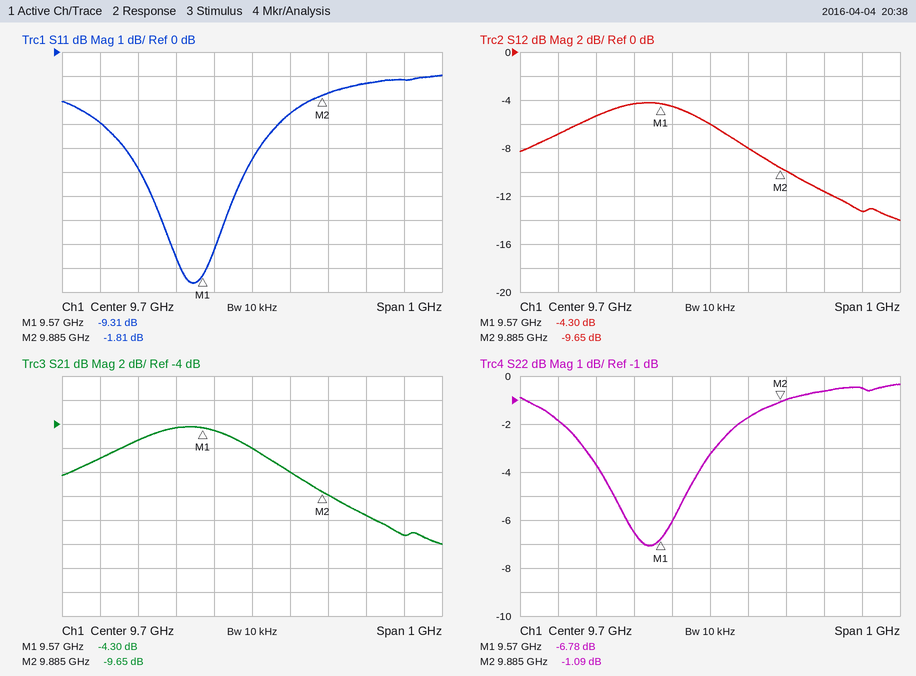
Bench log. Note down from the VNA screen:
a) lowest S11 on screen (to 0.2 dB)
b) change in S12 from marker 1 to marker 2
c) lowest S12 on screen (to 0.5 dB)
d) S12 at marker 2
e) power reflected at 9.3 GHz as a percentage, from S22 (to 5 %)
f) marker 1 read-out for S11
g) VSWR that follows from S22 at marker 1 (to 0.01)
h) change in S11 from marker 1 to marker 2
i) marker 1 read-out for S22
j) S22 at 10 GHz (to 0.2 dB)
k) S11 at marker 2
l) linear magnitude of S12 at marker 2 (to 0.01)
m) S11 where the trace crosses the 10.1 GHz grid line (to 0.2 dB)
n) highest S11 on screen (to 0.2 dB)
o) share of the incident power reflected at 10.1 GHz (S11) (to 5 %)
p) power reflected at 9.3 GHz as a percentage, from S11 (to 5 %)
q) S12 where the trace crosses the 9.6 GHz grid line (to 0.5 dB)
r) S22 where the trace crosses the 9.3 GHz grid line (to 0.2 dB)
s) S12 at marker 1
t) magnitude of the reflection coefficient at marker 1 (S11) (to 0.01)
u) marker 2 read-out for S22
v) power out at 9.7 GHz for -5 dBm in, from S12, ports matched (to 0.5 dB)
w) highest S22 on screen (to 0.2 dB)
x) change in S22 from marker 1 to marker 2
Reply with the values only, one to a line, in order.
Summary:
-9.6 dB
-5.35 dB
-14.0 dB
-9.65 dB
65 %
-9.31 dB
2.69
7.50 dB
-6.78 dB
-0.6 dB
-1.81 dB
0.33
-1.2 dB
-1.0 dB
75 %
50 %
-4.5 dB
-1.8 dB
-4.30 dB
0.34
-1.09 dB
-11.0 dBm
-0.4 dB
5.69 dB
